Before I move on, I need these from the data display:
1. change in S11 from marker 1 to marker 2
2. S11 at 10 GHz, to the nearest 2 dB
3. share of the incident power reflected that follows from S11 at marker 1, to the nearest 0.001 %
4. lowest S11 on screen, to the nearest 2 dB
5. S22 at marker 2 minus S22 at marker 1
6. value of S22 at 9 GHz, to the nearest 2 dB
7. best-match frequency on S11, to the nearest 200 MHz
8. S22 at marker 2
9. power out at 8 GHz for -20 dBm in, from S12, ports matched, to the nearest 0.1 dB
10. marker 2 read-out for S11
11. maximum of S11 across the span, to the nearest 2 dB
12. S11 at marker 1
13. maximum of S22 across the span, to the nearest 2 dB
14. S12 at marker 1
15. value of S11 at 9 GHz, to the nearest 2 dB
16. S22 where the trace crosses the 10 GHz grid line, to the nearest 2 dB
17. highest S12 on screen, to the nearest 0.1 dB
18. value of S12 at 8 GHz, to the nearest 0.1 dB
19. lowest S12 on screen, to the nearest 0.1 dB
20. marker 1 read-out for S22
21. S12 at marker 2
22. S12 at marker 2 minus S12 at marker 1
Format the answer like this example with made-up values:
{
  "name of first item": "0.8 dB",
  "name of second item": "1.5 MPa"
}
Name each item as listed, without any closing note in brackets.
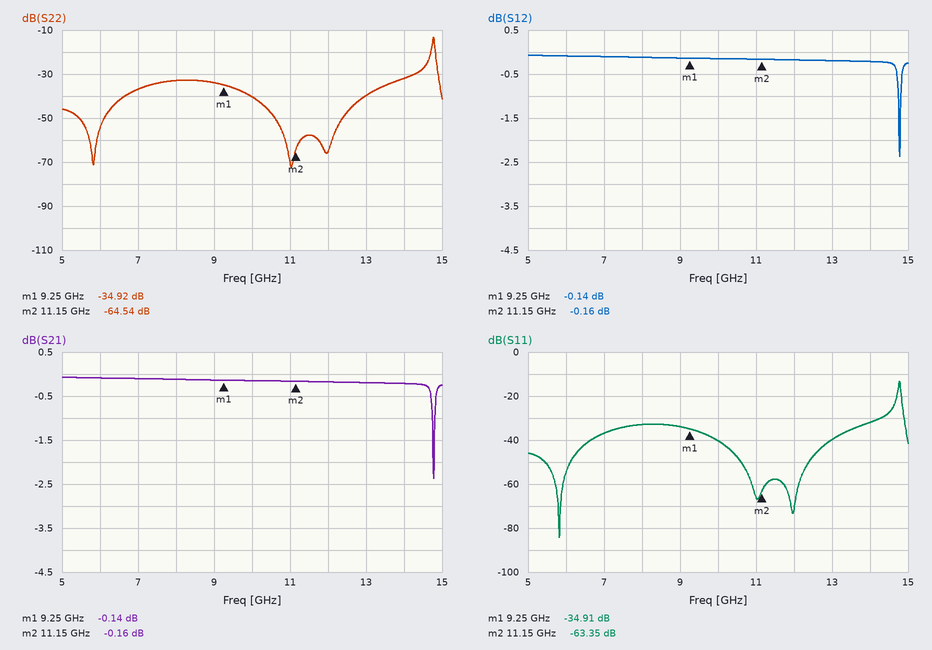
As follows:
{
  "change in S11 from marker 1 to marker 2": "-28.44 dB",
  "S11 at 10 GHz, to the nearest 2 dB": "-40 dB",
  "share of the incident power reflected that follows from S11 at marker 1, to the nearest 0.001 %": "0.032 %",
  "lowest S11 on screen, to the nearest 2 dB": "-84 dB",
  "S22 at marker 2 minus S22 at marker 1": "-29.62 dB",
  "value of S22 at 9 GHz, to the nearest 2 dB": "-34 dB",
  "best-match frequency on S11, to the nearest 200 MHz": "5.8 GHz",
  "S22 at marker 2": "-64.54 dB",
  "power out at 8 GHz for -20 dBm in, from S12, ports matched, to the nearest 0.1 dB": "-20.1 dBm",
  "marker 2 read-out for S11": "-63.35 dB",
  "maximum of S11 across the span, to the nearest 2 dB": "-14 dB",
  "S11 at marker 1": "-34.91 dB",
  "maximum of S22 across the span, to the nearest 2 dB": "-14 dB",
  "S12 at marker 1": "-0.14 dB",
  "value of S11 at 9 GHz, to the nearest 2 dB": "-34 dB",
  "S22 where the trace crosses the 10 GHz grid line, to the nearest 2 dB": "-40 dB",
  "highest S12 on screen, to the nearest 0.1 dB": "-0.1 dB",
  "value of S12 at 8 GHz, to the nearest 0.1 dB": "-0.1 dB",
  "lowest S12 on screen, to the nearest 0.1 dB": "-2.4 dB",
  "marker 1 read-out for S22": "-34.92 dB",
  "S12 at marker 2": "-0.16 dB",
  "S12 at marker 2 minus S12 at marker 1": "-0.02 dB"
}
